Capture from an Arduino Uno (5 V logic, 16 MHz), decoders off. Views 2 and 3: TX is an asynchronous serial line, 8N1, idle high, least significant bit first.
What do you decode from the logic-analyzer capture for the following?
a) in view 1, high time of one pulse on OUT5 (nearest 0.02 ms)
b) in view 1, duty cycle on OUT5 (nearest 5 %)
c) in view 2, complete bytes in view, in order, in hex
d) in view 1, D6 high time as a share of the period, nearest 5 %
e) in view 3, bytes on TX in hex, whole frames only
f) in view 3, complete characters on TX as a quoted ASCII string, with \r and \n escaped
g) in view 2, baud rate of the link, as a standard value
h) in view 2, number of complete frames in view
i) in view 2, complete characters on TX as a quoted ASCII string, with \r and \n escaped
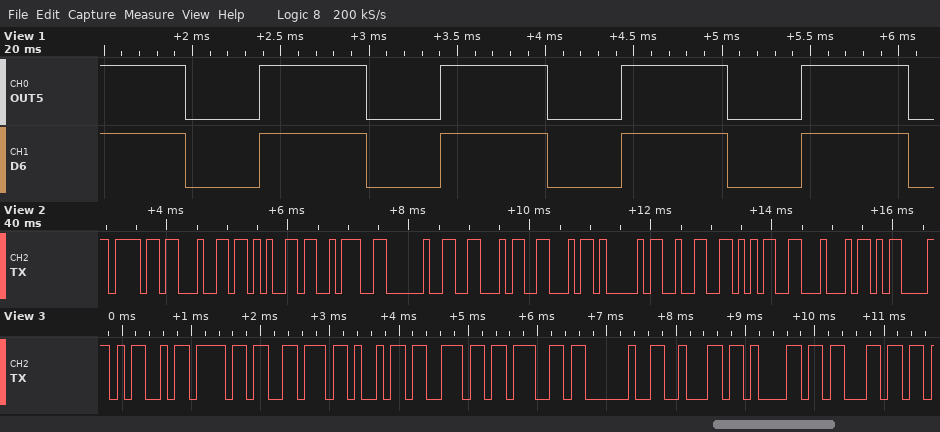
0.60 ms
60 %
6F 64 65 3A 20 46 46 41 32 35 44 0D
60 %
4D 6F 76 69 6E 67 20 62 61 63
"Moving bac"
9600 baud
12
"ode: FFA25D\r"
